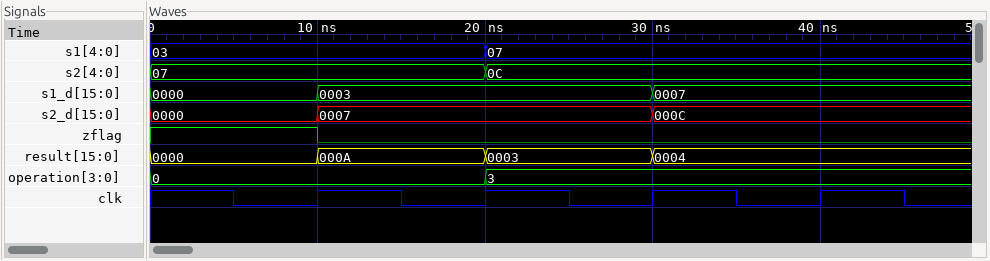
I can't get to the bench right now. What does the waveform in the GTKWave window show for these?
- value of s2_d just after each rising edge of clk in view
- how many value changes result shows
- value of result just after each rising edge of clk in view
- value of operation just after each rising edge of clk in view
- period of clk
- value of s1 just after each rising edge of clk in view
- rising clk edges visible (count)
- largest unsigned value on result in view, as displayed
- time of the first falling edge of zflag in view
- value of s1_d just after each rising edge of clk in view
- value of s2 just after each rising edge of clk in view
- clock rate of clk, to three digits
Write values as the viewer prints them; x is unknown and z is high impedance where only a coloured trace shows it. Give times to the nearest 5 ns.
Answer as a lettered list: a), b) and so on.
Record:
a) 0007, 0007, 000C, 000C
b) 3
c) 000A, 0003, 0004, 0004
d) 0, 3, 3, 3
e) 10 ns
f) 03, 07, 07, 07
g) 4
h) 000A
i) 10 ns
j) 0003, 0003, 0007, 0007
k) 07, 0C, 0C, 0C
l) 100 MHz
